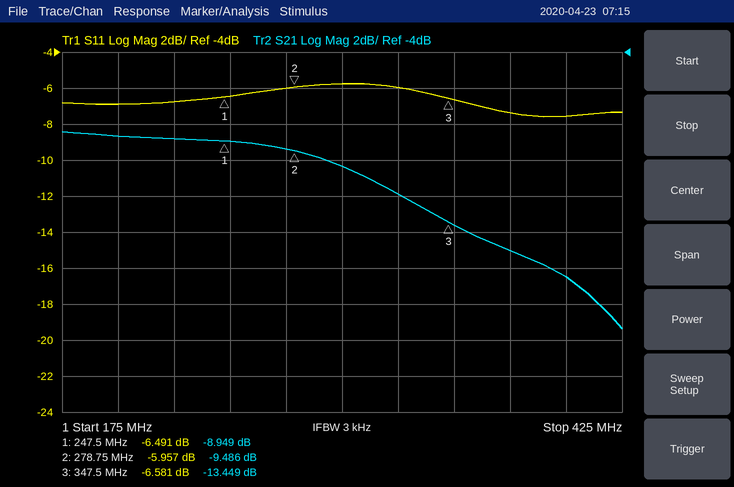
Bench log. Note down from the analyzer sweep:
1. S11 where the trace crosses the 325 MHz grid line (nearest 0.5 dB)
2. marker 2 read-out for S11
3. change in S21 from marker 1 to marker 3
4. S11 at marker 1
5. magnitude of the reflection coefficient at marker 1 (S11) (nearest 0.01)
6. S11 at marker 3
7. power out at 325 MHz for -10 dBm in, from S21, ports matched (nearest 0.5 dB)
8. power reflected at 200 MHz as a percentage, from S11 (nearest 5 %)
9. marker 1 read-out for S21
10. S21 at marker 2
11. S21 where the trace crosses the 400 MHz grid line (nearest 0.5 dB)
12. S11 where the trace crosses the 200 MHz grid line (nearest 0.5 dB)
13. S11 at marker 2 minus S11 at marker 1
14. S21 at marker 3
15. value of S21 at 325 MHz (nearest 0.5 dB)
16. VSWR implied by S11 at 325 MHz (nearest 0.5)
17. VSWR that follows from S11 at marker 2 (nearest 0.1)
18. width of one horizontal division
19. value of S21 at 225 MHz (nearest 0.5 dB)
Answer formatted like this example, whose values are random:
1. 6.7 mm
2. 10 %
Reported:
1. -6.0 dB
2. -5.957 dB
3. -4.500 dB
4. -6.491 dB
5. 0.47
6. -6.581 dB
7. -22.0 dBm
8. 20 %
9. -8.949 dB
10. -9.486 dB
11. -16.5 dB
12. -7.0 dB
13. 0.534 dB
14. -13.449 dB
15. -12.0 dB
16. 3.0
17. 3.0
18. 25 MHz
19. -9.0 dB
